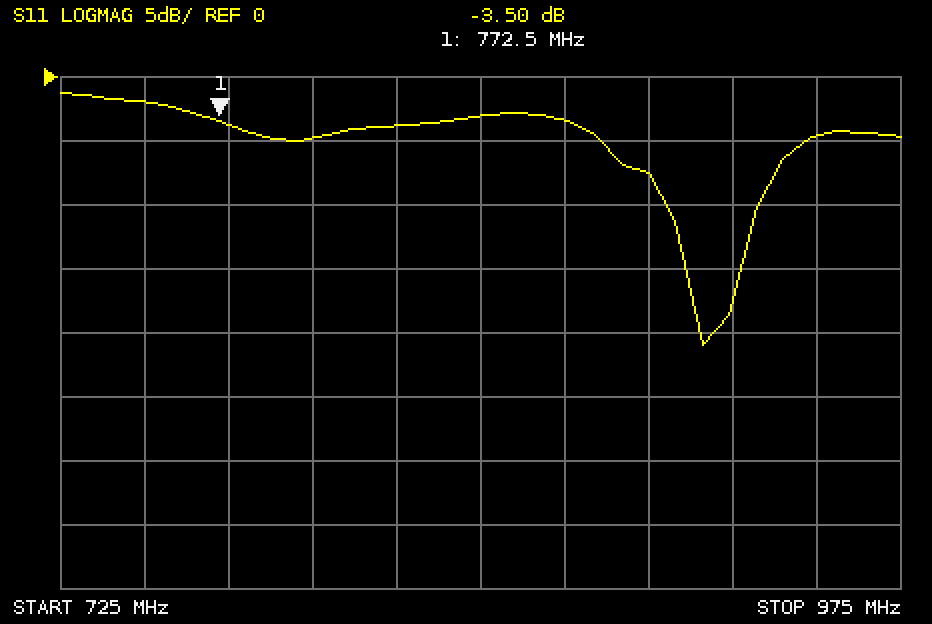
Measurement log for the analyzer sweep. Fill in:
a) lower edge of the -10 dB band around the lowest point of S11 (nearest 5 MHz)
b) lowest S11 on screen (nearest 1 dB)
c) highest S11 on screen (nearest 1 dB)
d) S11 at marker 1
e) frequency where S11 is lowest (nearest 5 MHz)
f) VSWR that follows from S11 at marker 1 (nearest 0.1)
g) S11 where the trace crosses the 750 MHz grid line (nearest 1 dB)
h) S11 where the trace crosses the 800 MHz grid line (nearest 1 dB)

905 MHz
-21 dB
-1 dB
-3.50 dB
915 MHz
5.0
-2 dB
-5 dB
